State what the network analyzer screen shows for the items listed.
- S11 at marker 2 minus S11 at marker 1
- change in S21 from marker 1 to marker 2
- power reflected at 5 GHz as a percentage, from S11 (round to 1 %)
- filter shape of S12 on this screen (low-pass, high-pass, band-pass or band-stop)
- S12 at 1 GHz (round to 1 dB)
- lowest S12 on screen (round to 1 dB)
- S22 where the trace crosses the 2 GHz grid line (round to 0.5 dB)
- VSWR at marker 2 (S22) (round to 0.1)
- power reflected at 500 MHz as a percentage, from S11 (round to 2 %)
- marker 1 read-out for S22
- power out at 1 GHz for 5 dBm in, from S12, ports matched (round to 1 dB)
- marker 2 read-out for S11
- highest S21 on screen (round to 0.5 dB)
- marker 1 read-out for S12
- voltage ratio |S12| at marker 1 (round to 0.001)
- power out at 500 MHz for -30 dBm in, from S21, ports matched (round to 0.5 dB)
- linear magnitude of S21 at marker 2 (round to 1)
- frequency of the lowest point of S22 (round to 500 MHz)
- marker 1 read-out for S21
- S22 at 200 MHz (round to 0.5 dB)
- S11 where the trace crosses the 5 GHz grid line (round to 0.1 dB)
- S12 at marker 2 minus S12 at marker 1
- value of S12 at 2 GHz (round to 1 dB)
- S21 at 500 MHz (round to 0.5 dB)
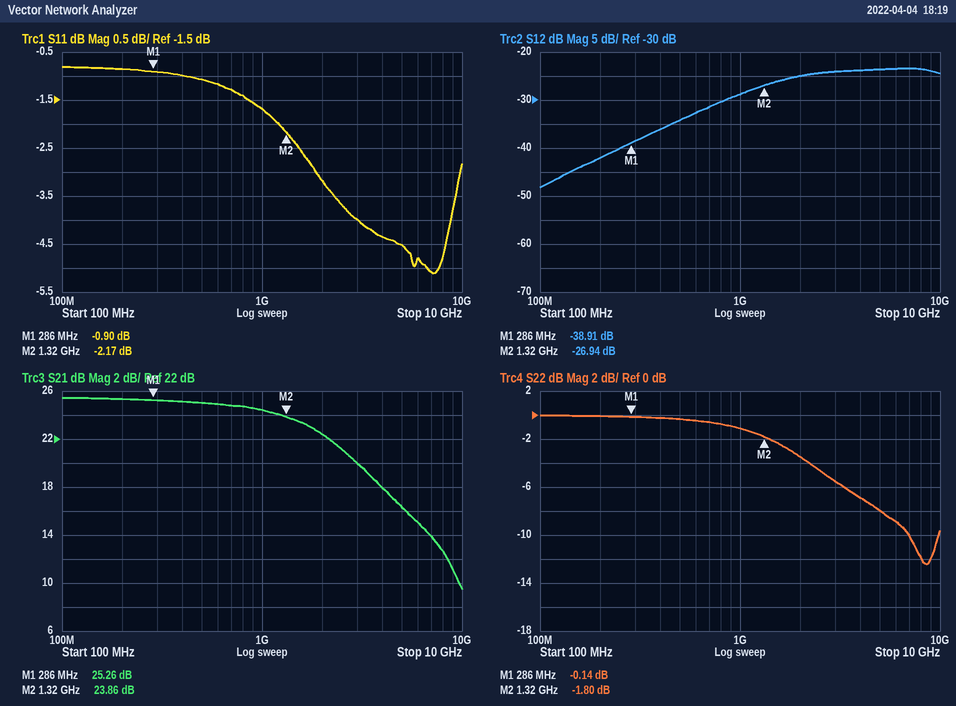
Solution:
-1.27 dB
-1.40 dB
35 %
high-pass
-29 dB
-48 dB
-3.5 dB
9.7
78 %
-0.14 dB
-24 dBm
-2.17 dB
25.5 dB
-38.91 dB
0.011
-5.0 dBm
16
8.5 GHz
25.26 dB
0.0 dB
-4.5 dB
11.97 dB
-25 dB
25.0 dB
